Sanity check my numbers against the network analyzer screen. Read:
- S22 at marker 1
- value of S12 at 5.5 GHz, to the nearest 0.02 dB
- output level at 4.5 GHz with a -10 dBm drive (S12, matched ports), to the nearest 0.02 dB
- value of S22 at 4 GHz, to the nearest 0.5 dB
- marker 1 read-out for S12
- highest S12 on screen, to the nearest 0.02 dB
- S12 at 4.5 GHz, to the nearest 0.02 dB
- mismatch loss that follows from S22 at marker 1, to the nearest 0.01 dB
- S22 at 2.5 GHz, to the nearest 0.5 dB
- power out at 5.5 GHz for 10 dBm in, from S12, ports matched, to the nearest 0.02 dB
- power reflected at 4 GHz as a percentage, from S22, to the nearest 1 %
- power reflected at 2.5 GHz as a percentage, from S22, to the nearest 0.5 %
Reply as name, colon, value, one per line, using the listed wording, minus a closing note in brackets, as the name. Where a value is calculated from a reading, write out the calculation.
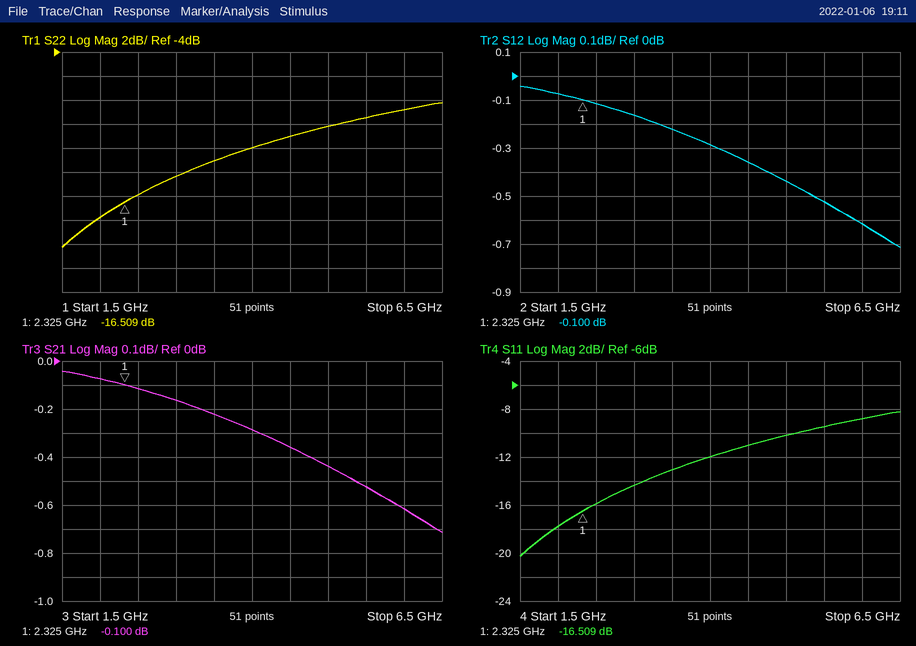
S22 at marker 1: -16.509 dB
value of S12 at 5.5 GHz, to the nearest 0.02 dB: -0.52 dB
output level at 4.5 GHz with a -10 dBm drive (S12, matched ports), to the nearest 0.02 dB: -10 dBm + (-0.36 dB) = -10.36 dBm
value of S22 at 4 GHz, to the nearest 0.5 dB: -12.0 dB
marker 1 read-out for S12: -0.100 dB
highest S12 on screen, to the nearest 0.02 dB: -0.04 dB
S12 at 4.5 GHz, to the nearest 0.02 dB: -0.36 dB
mismatch loss that follows from S22 at marker 1, to the nearest 0.01 dB: −10 log10(1 − 10^(-16.509/10)) ≈ 0.10 dB
S22 at 2.5 GHz, to the nearest 0.5 dB: -16.0 dB
power out at 5.5 GHz for 10 dBm in, from S12, ports matched, to the nearest 0.02 dB: 10 dBm + (-0.52 dB) = 9.48 dBm
power reflected at 4 GHz as a percentage, from S22, to the nearest 1 %: 10^(-12/10) ≈ 6 %
power reflected at 2.5 GHz as a percentage, from S22, to the nearest 0.5 %: 10^(-16/10) ≈ 2.5 %
